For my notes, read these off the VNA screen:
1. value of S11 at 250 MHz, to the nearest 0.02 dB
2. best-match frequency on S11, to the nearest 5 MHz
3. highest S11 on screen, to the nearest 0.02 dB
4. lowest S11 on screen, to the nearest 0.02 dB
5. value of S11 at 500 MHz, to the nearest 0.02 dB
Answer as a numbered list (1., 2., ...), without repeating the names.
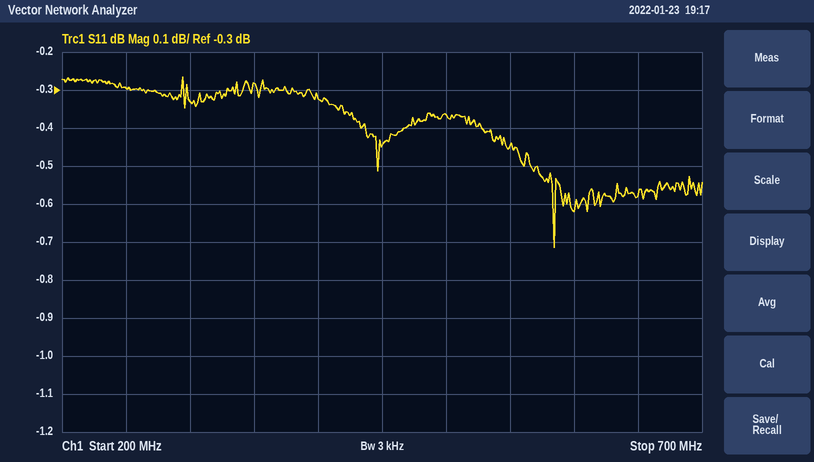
1. -0.30 dB
2. 585 MHz
3. -0.26 dB
4. -0.72 dB
5. -0.36 dB
